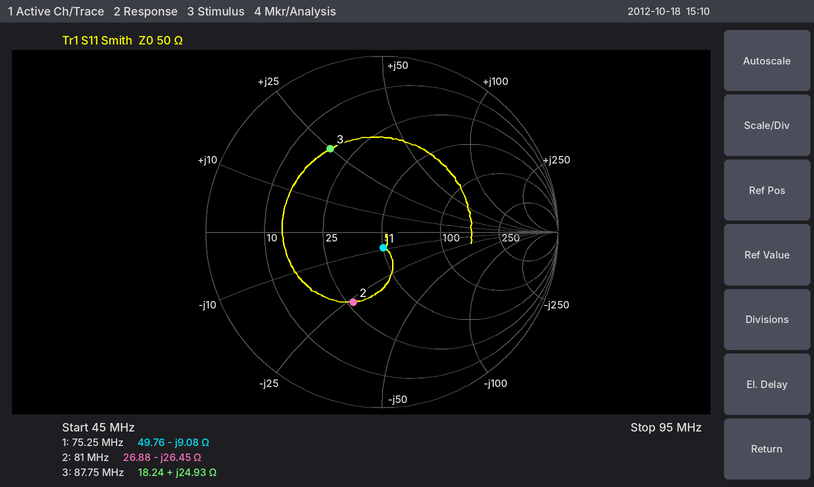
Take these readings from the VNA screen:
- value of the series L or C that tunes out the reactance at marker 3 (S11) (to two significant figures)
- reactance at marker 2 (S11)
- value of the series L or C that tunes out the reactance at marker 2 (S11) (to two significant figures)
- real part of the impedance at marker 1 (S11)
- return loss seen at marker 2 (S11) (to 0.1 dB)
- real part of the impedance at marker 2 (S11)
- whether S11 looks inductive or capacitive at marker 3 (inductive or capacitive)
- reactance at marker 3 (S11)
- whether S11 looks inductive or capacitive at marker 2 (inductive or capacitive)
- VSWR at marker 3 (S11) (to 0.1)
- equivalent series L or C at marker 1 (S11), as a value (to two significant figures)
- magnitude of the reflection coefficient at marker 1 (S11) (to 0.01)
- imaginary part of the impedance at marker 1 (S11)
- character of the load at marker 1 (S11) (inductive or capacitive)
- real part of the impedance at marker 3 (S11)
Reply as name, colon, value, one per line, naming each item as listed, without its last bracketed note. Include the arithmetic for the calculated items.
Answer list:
value of the series L or C that tunes out the reactance at marker 3 (S11): C = 1/(2π × 87.75 MHz × 24.93 Ω) ≈ 73 pF
reactance at marker 2: -26.45 Ω
value of the series L or C that tunes out the reactance at marker 2 (S11): L = 26.45 Ω/(2π × 81 MHz) ≈ 52 nH
real part of the impedance at marker 1: 49.76 Ω
return loss seen at marker 2 (S11): 7.3 dB
real part of the impedance at marker 2: 26.88 Ω
whether S11 looks inductive or capacitive at marker 3: inductive
reactance at marker 3: +24.93 Ω
whether S11 looks inductive or capacitive at marker 2: capacitive
VSWR at marker 3 (S11): 3.5
equivalent series L or C at marker 1 (S11), as a value: C = 1/(2π × 75.25 MHz × 9.08 Ω) ≈ 233 pF, so 230 pF to two significant figures
magnitude of the reflection coefficient at marker 1 (S11): 0.09
imaginary part of the impedance at marker 1: -9.08 Ω
character of the load at marker 1 (S11): capacitive
real part of the impedance at marker 3: 18.24 Ω
